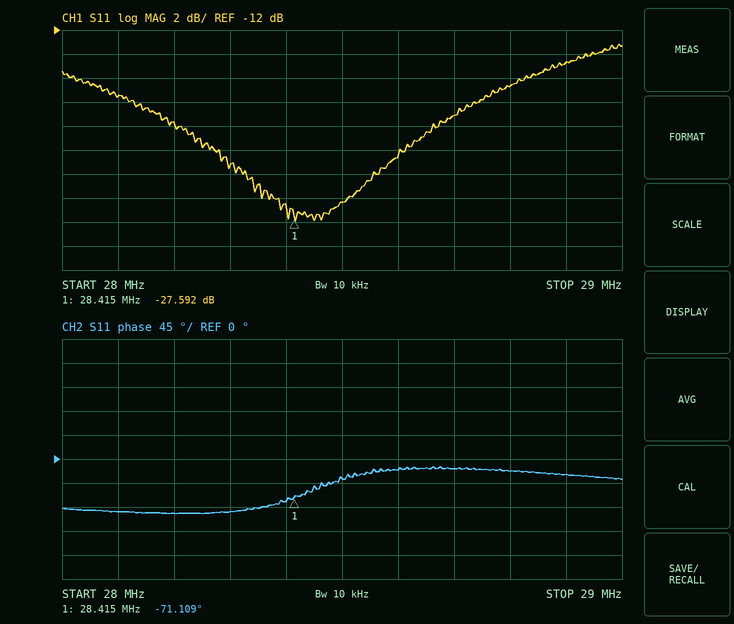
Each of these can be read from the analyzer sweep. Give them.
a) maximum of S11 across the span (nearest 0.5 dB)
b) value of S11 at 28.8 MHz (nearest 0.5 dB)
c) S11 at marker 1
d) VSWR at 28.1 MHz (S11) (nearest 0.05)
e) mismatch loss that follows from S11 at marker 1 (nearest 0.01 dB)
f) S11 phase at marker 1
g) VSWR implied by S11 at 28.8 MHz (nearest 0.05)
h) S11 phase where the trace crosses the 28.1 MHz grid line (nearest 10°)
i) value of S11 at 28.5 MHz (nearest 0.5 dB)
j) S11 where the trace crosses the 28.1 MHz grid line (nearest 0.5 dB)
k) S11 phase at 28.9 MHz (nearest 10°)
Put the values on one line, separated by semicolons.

-13.0 dB; -16.5 dB; -27.592 dB; 1.30; 0.01 dB; -71.109°; 1.35; -100°; -26.5 dB; -17.5 dB; -30°
